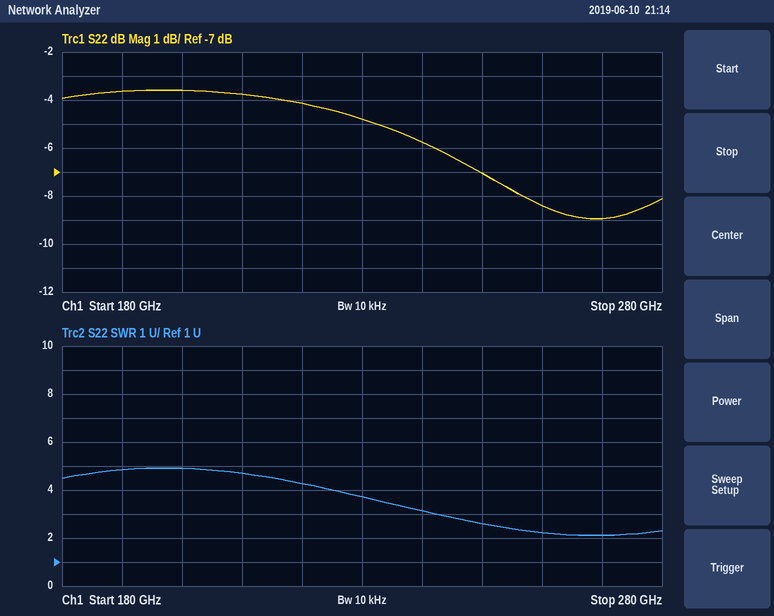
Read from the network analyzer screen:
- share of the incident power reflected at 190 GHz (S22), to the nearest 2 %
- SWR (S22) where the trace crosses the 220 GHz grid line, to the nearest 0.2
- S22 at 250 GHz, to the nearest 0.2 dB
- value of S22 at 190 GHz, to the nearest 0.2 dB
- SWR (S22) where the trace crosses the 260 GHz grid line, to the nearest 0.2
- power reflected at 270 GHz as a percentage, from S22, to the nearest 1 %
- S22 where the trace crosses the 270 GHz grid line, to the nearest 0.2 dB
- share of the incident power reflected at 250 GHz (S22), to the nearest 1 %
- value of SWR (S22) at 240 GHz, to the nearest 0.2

44 %
4.2
-7.0 dB
-3.6 dB
2.2
13 %
-9.0 dB
20 %
3.2
